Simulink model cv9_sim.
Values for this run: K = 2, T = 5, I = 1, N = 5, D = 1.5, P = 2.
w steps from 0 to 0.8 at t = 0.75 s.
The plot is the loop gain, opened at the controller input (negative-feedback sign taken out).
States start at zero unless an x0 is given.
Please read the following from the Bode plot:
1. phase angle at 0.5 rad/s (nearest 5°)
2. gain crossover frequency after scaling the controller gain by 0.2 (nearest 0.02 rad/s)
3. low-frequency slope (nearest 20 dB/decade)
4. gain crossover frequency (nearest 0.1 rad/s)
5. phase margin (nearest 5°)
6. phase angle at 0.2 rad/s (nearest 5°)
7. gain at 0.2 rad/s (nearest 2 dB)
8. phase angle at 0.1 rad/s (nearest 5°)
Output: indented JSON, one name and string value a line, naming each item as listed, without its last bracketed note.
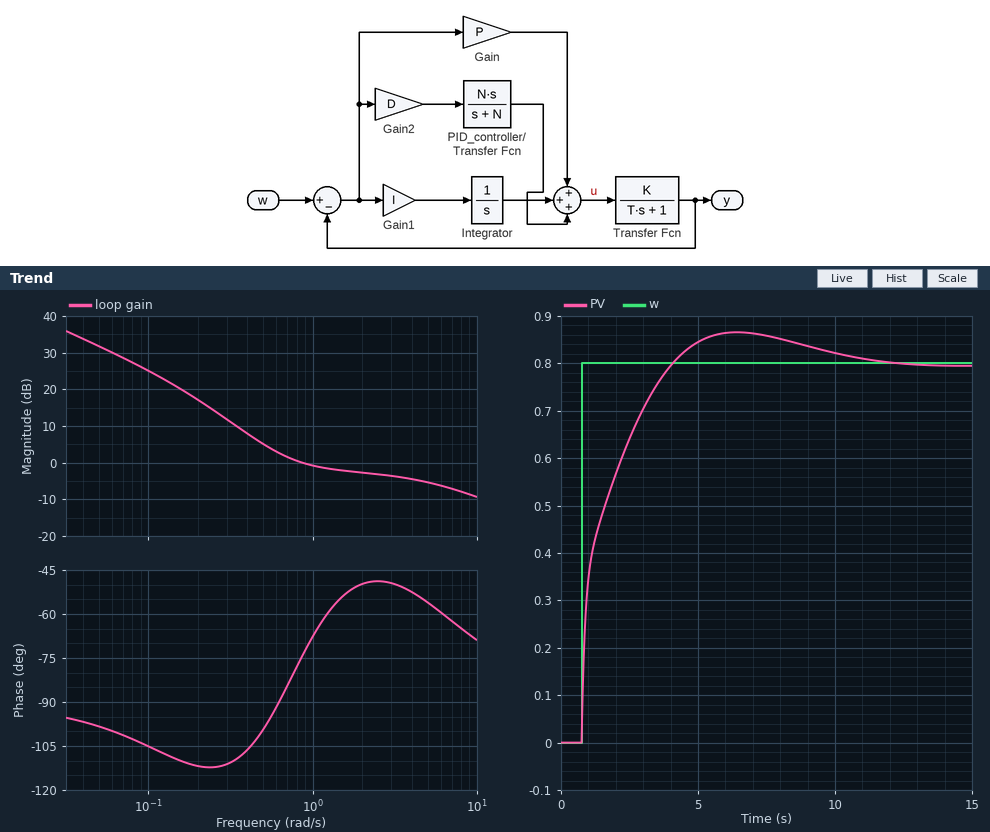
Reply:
{
  "phase angle at 0.5 rad/s": "-100°",
  "gain crossover frequency after scaling the controller gain by 0.2": "0.26 rad/s",
  "low-frequency slope": "-20 dB/decade",
  "gain crossover frequency": "0.9 rad/s",
  "phase margin": "105°",
  "phase angle at 0.2 rad/s": "-110°",
  "gain at 0.2 rad/s": "18 dB",
  "phase angle at 0.1 rad/s": "-105°"
}
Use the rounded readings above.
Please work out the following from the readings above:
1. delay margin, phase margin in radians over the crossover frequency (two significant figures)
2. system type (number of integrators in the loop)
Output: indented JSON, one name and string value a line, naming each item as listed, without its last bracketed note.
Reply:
{
  "delay margin, phase margin in radians over the crossover frequency": "2.0 s",
  "system type": "1"
}
